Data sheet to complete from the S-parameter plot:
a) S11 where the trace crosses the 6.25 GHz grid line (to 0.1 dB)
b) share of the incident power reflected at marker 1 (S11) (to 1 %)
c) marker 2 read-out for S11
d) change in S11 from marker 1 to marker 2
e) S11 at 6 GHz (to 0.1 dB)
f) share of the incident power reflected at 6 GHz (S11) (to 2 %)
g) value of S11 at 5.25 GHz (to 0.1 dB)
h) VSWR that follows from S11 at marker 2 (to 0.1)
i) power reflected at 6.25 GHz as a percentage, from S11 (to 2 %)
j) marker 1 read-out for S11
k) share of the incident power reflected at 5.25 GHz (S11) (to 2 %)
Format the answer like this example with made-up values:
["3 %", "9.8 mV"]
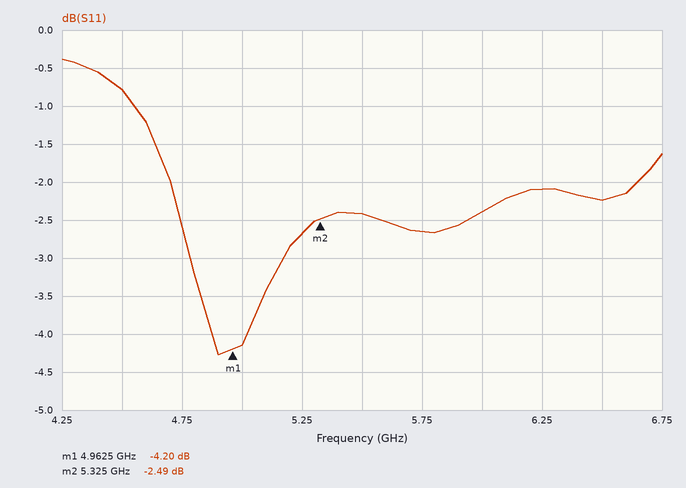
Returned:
["-2.1 dB", "38 %", "-2.49 dB", "1.71 dB", "-2.4 dB", "58 %", "-2.7 dB", "7.0", "62 %", "-4.20 dB", "54 %"]
